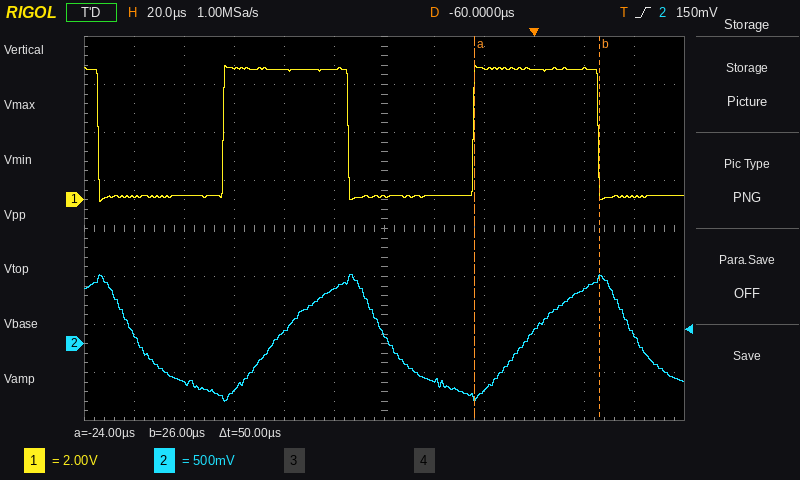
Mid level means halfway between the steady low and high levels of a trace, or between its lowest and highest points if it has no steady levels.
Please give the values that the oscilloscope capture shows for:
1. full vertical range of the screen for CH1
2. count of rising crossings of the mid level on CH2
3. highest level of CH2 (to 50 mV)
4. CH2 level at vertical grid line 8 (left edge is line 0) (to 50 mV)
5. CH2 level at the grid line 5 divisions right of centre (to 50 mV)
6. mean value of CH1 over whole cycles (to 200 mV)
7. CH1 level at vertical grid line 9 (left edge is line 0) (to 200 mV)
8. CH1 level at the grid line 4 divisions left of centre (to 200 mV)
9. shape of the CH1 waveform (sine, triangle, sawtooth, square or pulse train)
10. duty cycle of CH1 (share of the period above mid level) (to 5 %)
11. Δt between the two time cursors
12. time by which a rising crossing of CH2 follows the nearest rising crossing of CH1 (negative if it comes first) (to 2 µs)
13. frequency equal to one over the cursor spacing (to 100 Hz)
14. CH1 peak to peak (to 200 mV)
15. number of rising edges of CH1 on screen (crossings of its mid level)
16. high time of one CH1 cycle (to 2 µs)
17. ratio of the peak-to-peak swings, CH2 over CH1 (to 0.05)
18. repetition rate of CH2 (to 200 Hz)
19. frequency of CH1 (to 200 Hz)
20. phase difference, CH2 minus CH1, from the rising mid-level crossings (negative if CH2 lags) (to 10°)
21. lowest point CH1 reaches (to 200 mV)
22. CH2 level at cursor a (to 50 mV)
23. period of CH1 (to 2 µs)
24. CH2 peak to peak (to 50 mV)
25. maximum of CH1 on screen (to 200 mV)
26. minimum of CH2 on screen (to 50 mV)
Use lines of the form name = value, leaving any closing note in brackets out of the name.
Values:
full vertical range of the screen for CH1 = 16 V
count of rising crossings of the mid level on CH2 = 2
highest level of CH2 = 700 mV
CH2 level at vertical grid line 8 (left edge is line 0) = -500 mV
CH2 level at the grid line 5 divisions right of centre = 100 mV
mean value of CH1 over whole cycles = 2.8 V
CH1 level at vertical grid line 9 (left edge is line 0) = 5.4 V
CH1 level at the grid line 4 divisions left of centre = 200 mV
shape of the CH1 waveform = square
duty cycle of CH1 (share of the period above mid level) = 50 %
Δt between the two time cursors = 50 µs
time by which a rising crossing of CH2 follows the nearest rising crossing of CH1 (negative if it comes first) = +22 µs
frequency equal to one over the cursor spacing = 20.0 kHz
CH1 peak to peak = 5.6 V
number of rising edges of CH1 on screen = 2
high time of one CH1 cycle = 50 µs
ratio of the peak-to-peak swings, CH2 over CH1 = 0.25
repetition rate of CH2 = 10.0 kHz
frequency of CH1 = 10.0 kHz
phase difference, CH2 minus CH1, from the rising mid-level crossings (negative if CH2 lags) = -80°
lowest point CH1 reaches = 0.0 V
CH2 level at cursor a = -550 mV
period of CH1 = 100 µs
CH2 peak to peak = 1.30 V
maximum of CH1 on screen = 5.6 V
minimum of CH2 on screen = -600 mV
